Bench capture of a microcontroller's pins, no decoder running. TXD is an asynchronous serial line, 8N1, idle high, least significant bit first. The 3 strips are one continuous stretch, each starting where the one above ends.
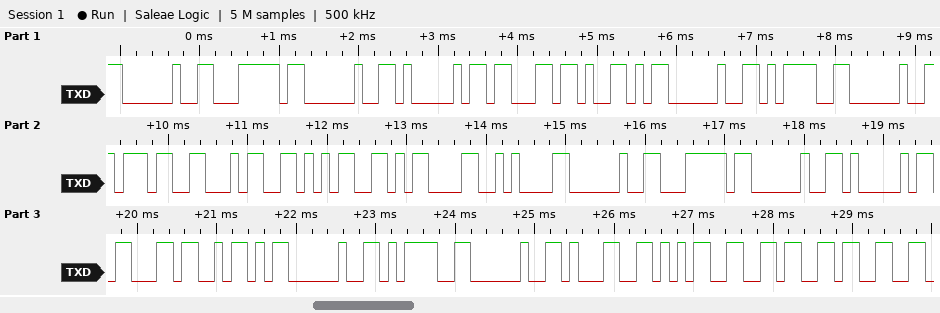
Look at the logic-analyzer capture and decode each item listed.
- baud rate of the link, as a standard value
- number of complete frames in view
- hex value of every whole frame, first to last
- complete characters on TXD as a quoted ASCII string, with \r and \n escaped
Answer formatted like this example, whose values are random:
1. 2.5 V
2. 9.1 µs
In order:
1. 9600 baud
2. 27
3. 20 7C 20 41 63 59 20 3D 20 37 34 35 0D 0A 20 7C 20 41 63 5A 20 3D 20 31 35 36 33
4. " | AcY = 745\r\n | AcZ = 1563"
